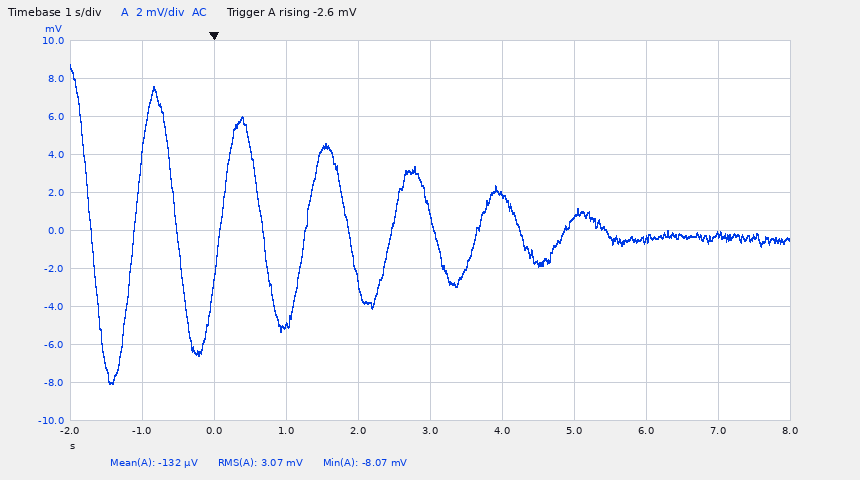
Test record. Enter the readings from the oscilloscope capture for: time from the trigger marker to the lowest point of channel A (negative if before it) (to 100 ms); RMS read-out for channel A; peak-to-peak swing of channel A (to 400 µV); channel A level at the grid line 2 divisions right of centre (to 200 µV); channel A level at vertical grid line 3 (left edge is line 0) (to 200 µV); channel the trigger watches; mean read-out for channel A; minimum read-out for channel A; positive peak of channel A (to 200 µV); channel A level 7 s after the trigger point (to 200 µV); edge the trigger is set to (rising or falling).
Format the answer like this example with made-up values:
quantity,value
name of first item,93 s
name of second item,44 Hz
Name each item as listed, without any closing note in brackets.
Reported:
quantity,value
time from the trigger marker to the lowest point of channel A (negative if before it),-1.4 s
RMS read-out for channel A,3.07 mV
peak-to-peak swing of channel A,16.8 mV
channel A level at the grid line 2 divisions right of centre,600 µV
channel A level at vertical grid line 3 (left edge is line 0),-5.0 mV
channel the trigger watches,channel A
mean read-out for channel A,-132 µV
minimum read-out for channel A,-8.07 mV
positive peak of channel A,8.8 mV
channel A level 7 s after the trigger point,-200 µV
edge the trigger is set to,rising
